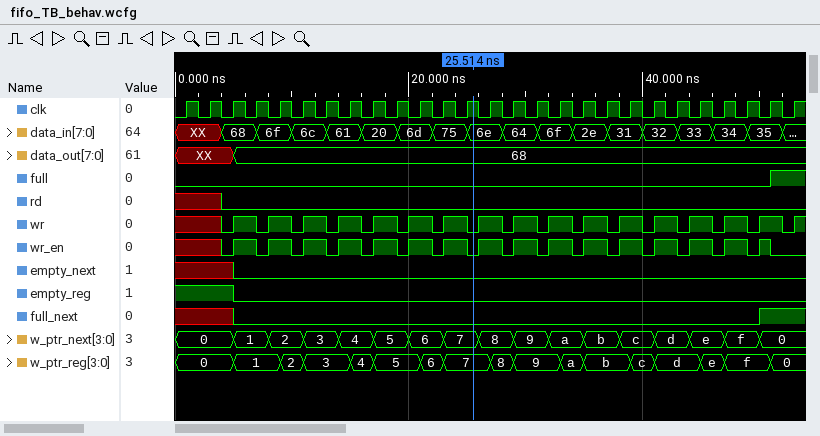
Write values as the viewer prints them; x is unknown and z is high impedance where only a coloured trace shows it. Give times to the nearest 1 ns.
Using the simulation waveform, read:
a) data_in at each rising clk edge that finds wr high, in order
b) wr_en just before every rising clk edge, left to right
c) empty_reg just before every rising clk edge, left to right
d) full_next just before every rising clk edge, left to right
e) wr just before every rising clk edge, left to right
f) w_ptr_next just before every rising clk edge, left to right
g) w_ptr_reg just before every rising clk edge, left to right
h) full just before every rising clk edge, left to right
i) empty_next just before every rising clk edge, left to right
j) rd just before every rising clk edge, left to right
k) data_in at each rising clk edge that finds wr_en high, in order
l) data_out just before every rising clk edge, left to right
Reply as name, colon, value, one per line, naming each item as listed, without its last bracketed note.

data_in at each rising clk edge that finds wr high, in order: 68, 6f, 6c, 61, 20, 6d, 75, 6e, 64, 6f, 2e, 31, 32, 33, 34, 35
wr_en just before every rising clk edge, left to right: x x 0 1 1 0 1 1 0 1 1 0 1 1 0 1 1 0 1 1 0 1 1 0 1 1 0
empty_reg just before every rising clk edge, left to right: 1 1 1 0 0 0 0 0 0 0 0 0 0 0 0 0 0 0 0 0 0 0 0 0 0 0 0
full_next just before every rising clk edge, left to right: x x x 0 0 0 0 0 0 0 0 0 0 0 0 0 0 0 0 0 0 0 0 0 0 1 1
wr just before every rising clk edge, left to right: x x 0 1 1 0 1 1 0 1 1 0 1 1 0 1 1 0 1 1 0 1 1 0 1 1 0
w_ptr_next just before every rising clk edge, left to right: 0, 0, 0, 1, 2, 2, 3, 4, 4, 5, 6, 6, 7, 8, 8, 9, a, a, b, c, c, d, e, e, f, 0, 0
w_ptr_reg just before every rising clk edge, left to right: 0, 0, 0, 1, 1, 2, 3, 3, 4, 5, 5, 6, 7, 7, 8, 9, 9, a, b, b, c, d, d, e, f, f, 0
full just before every rising clk edge, left to right: 0 0 0 0 0 0 0 0 0 0 0 0 0 0 0 0 0 0 0 0 0 0 0 0 0 0 1
empty_next just before every rising clk edge, left to right: x x x 0 0 0 0 0 0 0 0 0 0 0 0 0 0 0 0 0 0 0 0 0 0 0 0
rd just before every rising clk edge, left to right: x x 0 0 0 0 0 0 0 0 0 0 0 0 0 0 0 0 0 0 0 0 0 0 0 0 0
data_in at each rising clk edge that finds wr_en high, in order: 68, 6f, 6c, 61, 20, 6d, 75, 6e, 64, 6f, 2e, 31, 32, 33, 34, 35
data_out just before every rising clk edge, left to right: XX, XX, XX, 68, 68, 68, 68, 68, 68, 68, 68, 68, 68, 68, 68, 68, 68, 68, 68, 68, 68, 68, 68, 68, 68, 68, 68
